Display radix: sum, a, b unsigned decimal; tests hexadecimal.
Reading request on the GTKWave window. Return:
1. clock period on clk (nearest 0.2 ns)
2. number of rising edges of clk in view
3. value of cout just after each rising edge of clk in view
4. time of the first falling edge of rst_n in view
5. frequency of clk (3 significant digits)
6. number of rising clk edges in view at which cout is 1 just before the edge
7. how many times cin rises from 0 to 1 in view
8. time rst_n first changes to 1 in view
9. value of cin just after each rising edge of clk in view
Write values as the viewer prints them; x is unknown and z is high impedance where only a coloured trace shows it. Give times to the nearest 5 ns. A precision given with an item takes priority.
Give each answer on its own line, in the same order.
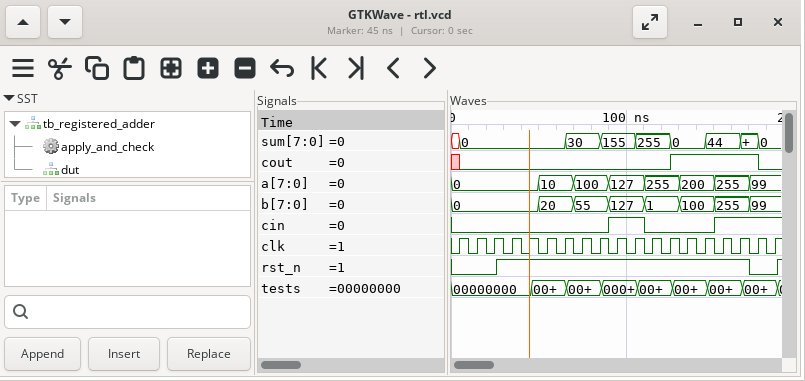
10 ns
19
0 0 0 0 0 0 0 0 0 0 0 0 1 1 1 1 1 0 0
170 ns
100 MHz
5
2
25 ns
0 0 0 0 0 0 0 0 0 1 1 0 0 0 0 1 1 1 1
